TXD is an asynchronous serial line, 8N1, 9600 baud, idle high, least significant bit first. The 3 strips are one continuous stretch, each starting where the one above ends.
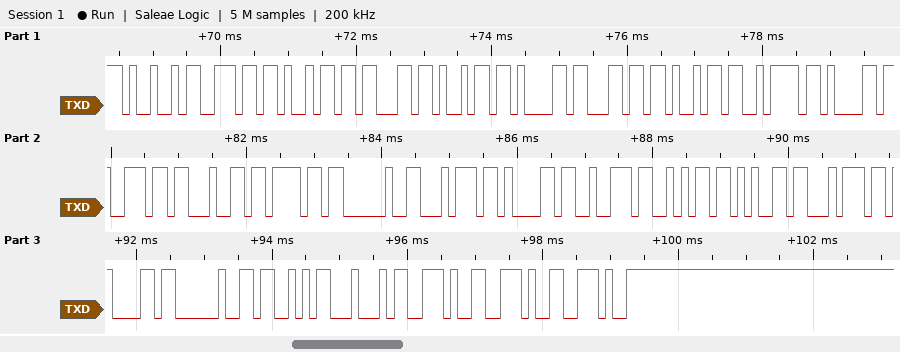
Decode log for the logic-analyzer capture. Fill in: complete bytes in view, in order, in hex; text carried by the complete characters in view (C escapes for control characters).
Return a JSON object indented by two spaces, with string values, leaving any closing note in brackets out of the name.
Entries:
{
  "complete bytes in view, in order, in hex": "0x49 0x6E 0x69 0x63 0x69 0x61 0x6C 0x69 0x7A 0x61 0x6E 0x64 0x6F 0x20 0x74 0x61 0x72 0x6A 0x65 0x74 0x61 0x20 0x53 0x44 0x2E 0x2E 0x2E",
  "text carried by the complete characters in view": "\"Inicializando tarjeta SD...\""
}
